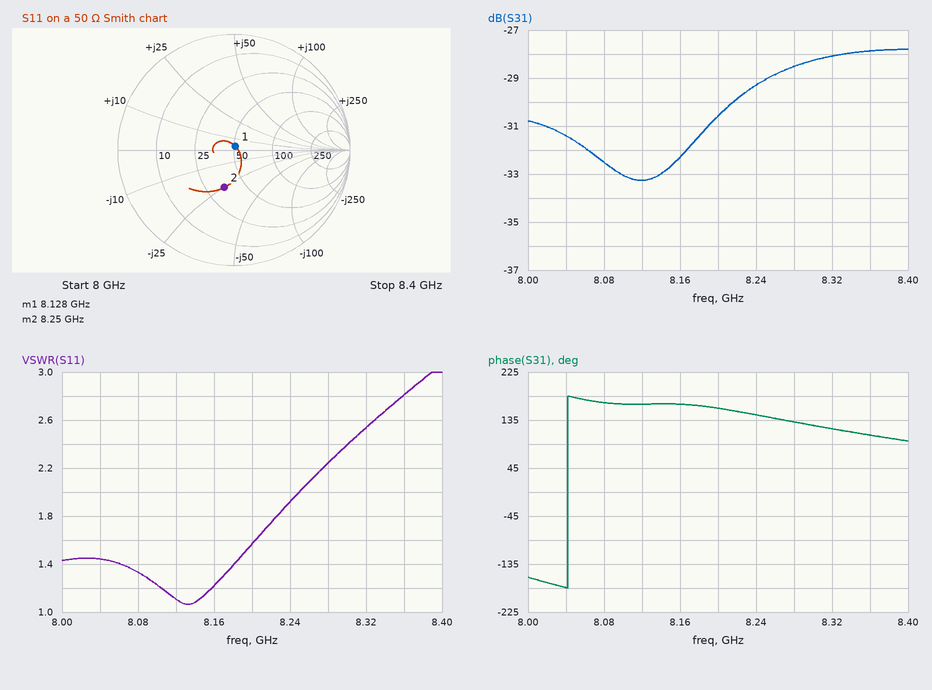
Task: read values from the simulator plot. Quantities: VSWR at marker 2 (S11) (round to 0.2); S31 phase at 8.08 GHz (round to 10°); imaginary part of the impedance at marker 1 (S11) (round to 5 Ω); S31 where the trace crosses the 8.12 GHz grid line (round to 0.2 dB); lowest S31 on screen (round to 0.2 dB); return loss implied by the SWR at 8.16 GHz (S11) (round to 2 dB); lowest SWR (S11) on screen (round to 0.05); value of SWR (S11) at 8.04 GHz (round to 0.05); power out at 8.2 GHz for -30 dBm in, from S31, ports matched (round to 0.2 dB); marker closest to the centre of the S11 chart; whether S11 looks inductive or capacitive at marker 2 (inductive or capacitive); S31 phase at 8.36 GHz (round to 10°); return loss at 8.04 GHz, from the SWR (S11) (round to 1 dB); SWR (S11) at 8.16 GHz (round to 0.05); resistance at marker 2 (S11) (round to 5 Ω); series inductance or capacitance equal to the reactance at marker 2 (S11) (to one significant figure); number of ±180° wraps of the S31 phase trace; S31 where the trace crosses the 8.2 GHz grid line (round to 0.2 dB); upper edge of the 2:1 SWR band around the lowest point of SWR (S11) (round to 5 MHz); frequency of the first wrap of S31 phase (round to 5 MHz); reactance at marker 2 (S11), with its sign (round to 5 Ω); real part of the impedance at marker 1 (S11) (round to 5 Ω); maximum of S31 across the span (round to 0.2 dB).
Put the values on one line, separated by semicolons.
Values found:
2.0; 170°; +5 Ω; -33.2 dB; -33.2 dB; 20 dB; 1.05; 1.45; -60.6 dBm; marker 1; capacitive; 110°; 15 dB; 1.20; 35 Ω; 800 fF; 1; -30.6 dB; 8.250 GHz; 8.040 GHz; -25 Ω; 50 Ω; -27.8 dB
